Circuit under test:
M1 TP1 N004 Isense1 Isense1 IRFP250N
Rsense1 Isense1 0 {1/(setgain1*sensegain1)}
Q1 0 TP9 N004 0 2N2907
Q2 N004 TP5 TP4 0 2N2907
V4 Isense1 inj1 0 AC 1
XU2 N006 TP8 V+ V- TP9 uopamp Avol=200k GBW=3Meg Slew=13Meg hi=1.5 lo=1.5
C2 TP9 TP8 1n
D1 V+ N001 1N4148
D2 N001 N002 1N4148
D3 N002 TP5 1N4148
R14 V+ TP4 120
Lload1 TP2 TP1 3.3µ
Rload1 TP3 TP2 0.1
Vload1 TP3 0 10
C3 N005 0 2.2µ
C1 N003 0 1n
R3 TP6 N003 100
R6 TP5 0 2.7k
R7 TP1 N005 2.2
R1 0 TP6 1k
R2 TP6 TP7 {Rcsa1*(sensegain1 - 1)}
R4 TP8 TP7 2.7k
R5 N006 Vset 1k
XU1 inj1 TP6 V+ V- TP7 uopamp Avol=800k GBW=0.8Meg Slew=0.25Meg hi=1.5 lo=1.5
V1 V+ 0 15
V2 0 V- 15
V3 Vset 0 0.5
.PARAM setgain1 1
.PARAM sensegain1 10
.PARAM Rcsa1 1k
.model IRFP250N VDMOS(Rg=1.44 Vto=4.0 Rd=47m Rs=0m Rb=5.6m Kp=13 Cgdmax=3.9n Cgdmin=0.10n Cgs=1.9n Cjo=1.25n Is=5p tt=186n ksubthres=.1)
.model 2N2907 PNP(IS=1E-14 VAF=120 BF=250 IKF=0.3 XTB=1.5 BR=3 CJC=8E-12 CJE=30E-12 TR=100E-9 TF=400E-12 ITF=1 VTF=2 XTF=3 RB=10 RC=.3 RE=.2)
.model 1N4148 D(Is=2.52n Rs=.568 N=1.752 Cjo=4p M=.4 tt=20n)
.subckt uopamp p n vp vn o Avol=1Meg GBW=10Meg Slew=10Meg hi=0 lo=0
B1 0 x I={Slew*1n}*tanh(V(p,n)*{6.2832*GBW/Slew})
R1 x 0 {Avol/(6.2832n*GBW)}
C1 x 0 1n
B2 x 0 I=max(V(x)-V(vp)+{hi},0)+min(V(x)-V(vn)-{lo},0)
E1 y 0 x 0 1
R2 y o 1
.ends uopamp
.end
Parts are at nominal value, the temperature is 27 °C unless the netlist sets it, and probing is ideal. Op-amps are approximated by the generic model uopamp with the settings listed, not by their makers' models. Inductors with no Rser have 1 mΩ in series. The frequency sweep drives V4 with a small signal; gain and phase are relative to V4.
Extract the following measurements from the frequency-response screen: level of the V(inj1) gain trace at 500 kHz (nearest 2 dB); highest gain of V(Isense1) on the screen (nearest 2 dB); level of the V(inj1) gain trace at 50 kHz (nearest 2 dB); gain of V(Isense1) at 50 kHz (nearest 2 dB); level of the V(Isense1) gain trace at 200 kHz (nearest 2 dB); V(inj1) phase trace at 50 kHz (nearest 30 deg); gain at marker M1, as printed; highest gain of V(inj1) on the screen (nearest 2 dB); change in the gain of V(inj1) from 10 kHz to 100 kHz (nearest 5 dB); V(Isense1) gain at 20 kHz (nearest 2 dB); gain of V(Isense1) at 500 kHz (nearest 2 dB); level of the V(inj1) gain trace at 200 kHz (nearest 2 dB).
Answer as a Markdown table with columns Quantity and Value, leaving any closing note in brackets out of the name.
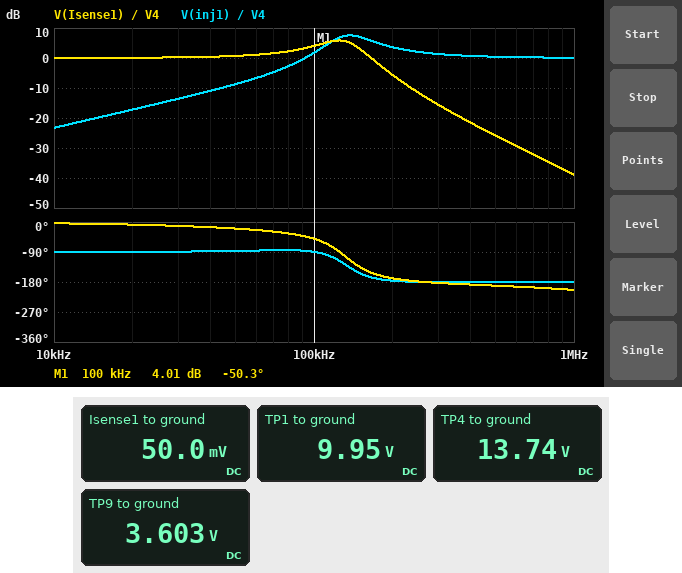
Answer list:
| Quantity | Value |
|---|---|
| level of the V(inj1) gain trace at 500 kHz | 0 dB |
| highest gain of V(Isense1) on the screen | 6 dB |
| level of the V(inj1) gain trace at 50 kHz | -8 dB |
| gain of V(Isense1) at 50 kHz | 0 dB |
| level of the V(Isense1) gain trace at 200 kHz | -6 dB |
| V(inj1) phase trace at 50 kHz | -90 deg |
| gain at marker M1, as printed | 4.01 dB |
| highest gain of V(inj1) on the screen | 8 dB |
| change in the gain of V(inj1) from 10 kHz to 100 kHz | 25 dB |
| V(Isense1) gain at 20 kHz | 0 dB |
| gain of V(Isense1) at 500 kHz | -26 dB |
| level of the V(inj1) gain trace at 200 kHz | 4 dB |
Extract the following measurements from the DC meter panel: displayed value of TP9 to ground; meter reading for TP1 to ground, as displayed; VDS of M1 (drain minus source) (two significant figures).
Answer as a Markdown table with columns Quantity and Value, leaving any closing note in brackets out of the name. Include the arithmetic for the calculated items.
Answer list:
| Quantity | Value |
|---|---|
| displayed value of TP9 to ground | 3.603 V |
| meter reading for TP1 to ground, as displayed | 9.95 V |
| VDS of M1 (drain minus source) | 9.95 V - 50 mV = 9.9 V |
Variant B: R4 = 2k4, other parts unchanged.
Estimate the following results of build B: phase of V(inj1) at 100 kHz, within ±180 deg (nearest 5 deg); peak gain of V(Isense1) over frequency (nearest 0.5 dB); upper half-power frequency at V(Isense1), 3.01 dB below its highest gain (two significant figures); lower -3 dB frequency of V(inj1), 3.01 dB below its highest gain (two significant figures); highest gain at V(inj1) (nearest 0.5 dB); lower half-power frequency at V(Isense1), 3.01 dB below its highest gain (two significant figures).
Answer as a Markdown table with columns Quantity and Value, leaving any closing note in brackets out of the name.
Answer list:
| Quantity | Value |
|---|---|
| phase of V(inj1) at 100 kHz, within ±180 deg | -80 deg |
| peak gain of V(Isense1) over frequency | 7.0 dB |
| upper half-power frequency at V(Isense1), 3.01 dB below its highest gain | 160 kHz |
| lower -3 dB frequency of V(inj1), 3.01 dB below its highest gain | 120 kHz |
| highest gain at V(inj1) | 8.5 dB |
| lower half-power frequency at V(Isense1), 3.01 dB below its highest gain | 99 kHz |
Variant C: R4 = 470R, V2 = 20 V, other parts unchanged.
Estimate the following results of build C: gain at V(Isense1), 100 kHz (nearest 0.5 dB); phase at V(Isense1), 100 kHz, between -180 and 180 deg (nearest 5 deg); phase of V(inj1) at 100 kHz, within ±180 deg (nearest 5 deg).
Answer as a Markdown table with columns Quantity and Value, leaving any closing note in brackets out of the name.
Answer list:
| Quantity | Value |
|---|---|
| gain at V(Isense1), 100 kHz | 1.0 dB |
| phase at V(Isense1), 100 kHz, between -180 and 180 deg | -5 deg |
| phase of V(inj1) at 100 kHz, within ±180 deg | -45 deg |
